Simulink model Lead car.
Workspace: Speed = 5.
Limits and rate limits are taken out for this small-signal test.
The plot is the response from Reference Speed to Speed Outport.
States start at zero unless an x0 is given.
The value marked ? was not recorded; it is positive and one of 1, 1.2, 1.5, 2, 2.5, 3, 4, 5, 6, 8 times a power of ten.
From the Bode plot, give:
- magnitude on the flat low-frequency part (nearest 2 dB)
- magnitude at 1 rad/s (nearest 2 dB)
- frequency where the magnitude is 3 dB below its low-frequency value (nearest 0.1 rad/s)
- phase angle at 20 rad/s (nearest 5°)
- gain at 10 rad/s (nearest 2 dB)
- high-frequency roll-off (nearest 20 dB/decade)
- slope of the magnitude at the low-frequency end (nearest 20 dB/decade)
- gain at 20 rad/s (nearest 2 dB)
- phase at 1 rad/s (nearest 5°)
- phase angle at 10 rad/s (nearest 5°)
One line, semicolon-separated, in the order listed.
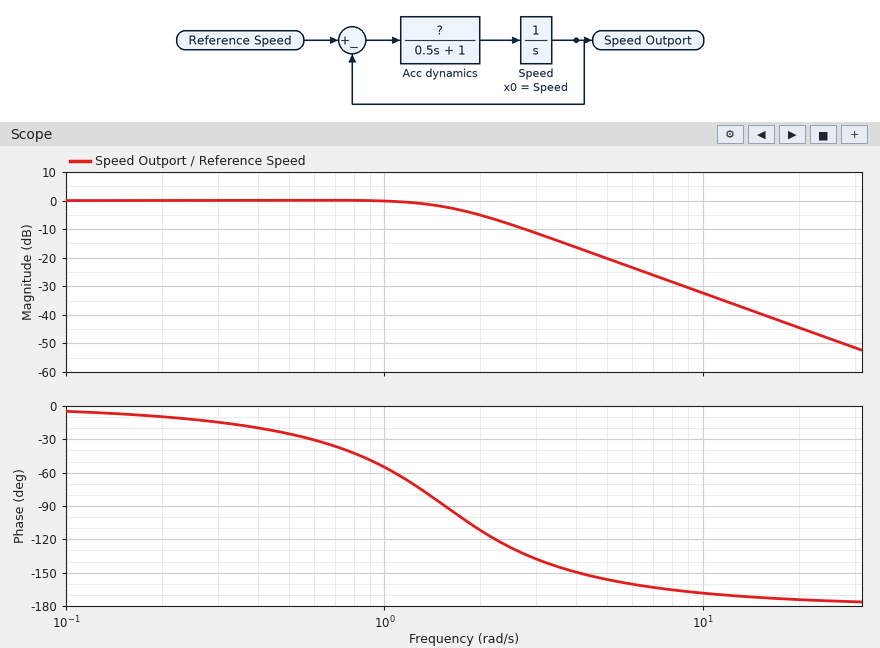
0 dB; 0 dB; 1.7 rad/s; -175°; -32 dB; -40 dB/decade; 0 dB/decade; -44 dB; -55°; -170°
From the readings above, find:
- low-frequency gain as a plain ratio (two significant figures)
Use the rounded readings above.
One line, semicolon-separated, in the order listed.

1.0
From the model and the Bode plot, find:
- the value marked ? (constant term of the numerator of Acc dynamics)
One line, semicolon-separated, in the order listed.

1.2
